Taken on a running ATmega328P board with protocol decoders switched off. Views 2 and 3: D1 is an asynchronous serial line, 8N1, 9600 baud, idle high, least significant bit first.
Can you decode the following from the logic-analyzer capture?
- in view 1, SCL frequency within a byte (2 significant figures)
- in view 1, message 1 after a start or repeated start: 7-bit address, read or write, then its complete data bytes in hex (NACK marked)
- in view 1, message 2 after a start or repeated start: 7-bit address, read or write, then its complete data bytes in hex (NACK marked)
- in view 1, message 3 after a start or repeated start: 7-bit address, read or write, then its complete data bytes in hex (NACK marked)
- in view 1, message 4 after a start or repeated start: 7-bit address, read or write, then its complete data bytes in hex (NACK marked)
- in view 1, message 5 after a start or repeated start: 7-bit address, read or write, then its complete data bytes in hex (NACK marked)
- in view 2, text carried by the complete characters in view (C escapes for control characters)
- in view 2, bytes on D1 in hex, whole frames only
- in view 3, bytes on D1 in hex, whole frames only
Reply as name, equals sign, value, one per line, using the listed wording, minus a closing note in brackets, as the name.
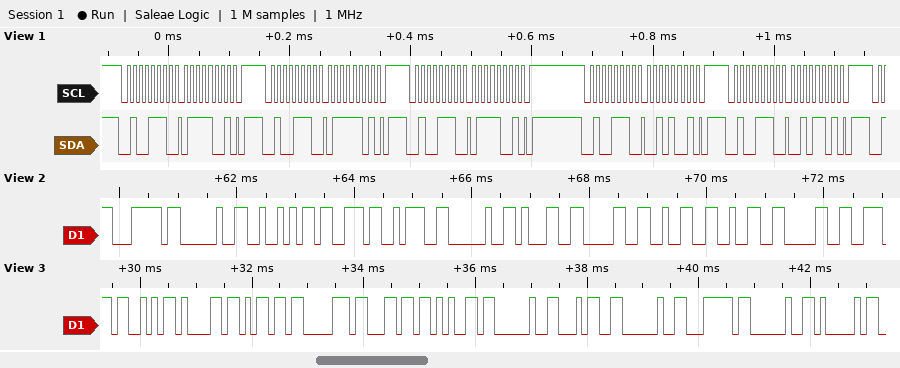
in view 1, SCL frequency within a byte = 100 kHz
in view 1, message 1 after a start or repeated start: 7-bit address, read or write, then its complete data bytes in hex = 0x27 write: 79
in view 1, message 2 after a start or repeated start: 7-bit address, read or write, then its complete data bytes in hex = 0x27 write: 7D
in view 1, message 3 after a start or repeated start: 7-bit address, read or write, then its complete data bytes in hex = 0x27 write: 79
in view 1, message 4 after a start or repeated start: 7-bit address, read or write, then its complete data bytes in hex = 0x27 write: 29
in view 1, message 5 after a start or repeated start: 7-bit address, read or write, then its complete data bytes in hex = 0x27 write: 2D
in view 2, text carried by the complete characters in view = "| Rs: 10220"
in view 2, bytes on D1 in hex, whole frames only = 7C 20 52 73 3A 20 31 30 32 32 30
in view 3, bytes on D1 in hex, whole frames only = 0x53 0x61 0x6D 0x70 0x6C 0x65 0x20 0x34 0x20 0x7C 0x20 0x41
